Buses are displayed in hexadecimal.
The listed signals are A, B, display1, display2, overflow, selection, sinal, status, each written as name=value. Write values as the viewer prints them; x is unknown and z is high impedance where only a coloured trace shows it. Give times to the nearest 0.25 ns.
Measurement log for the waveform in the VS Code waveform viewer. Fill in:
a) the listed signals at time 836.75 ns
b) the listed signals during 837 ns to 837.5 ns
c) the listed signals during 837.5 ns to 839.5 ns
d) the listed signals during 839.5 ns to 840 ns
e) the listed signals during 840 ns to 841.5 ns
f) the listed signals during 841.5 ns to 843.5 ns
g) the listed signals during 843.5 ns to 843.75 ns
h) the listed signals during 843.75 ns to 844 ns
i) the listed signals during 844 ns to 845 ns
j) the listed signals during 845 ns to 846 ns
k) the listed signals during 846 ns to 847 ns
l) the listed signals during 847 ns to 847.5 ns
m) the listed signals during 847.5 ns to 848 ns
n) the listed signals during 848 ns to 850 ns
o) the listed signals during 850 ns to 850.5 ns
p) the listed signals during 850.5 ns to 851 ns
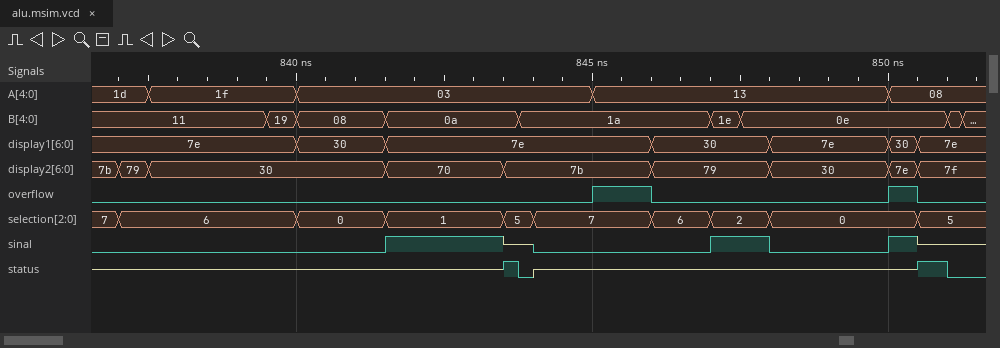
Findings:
A=1d, B=11, display1=7e, display2=7b, overflow=0, selection=7, sinal=0, status=z
A=1d, B=11, display1=7e, display2=79, overflow=0, selection=6, sinal=0, status=z
A=1f, B=11, display1=7e, display2=30, overflow=0, selection=6, sinal=0, status=z
A=1f, B=19, display1=7e, display2=30, overflow=0, selection=6, sinal=0, status=z
A=03, B=08, display1=30, display2=30, overflow=0, selection=0, sinal=0, status=z
A=03, B=0a, display1=7e, display2=70, overflow=0, selection=1, sinal=1, status=z
A=03, B=0a, display1=7e, display2=7b, overflow=0, selection=5, sinal=z, status=1
A=03, B=1a, display1=7e, display2=7b, overflow=0, selection=5, sinal=z, status=0
A=03, B=1a, display1=7e, display2=7b, overflow=0, selection=7, sinal=0, status=z
A=13, B=1a, display1=7e, display2=7b, overflow=1, selection=7, sinal=0, status=z
A=13, B=1a, display1=30, display2=79, overflow=0, selection=6, sinal=0, status=z
A=13, B=1e, display1=30, display2=79, overflow=0, selection=2, sinal=1, status=z
A=13, B=0e, display1=30, display2=79, overflow=0, selection=2, sinal=1, status=z
A=13, B=0e, display1=7e, display2=30, overflow=0, selection=0, sinal=0, status=z
A=08, B=0e, display1=30, display2=7e, overflow=1, selection=0, sinal=1, status=z
A=08, B=0e, display1=7e, display2=7f, overflow=0, selection=5, sinal=z, status=1
